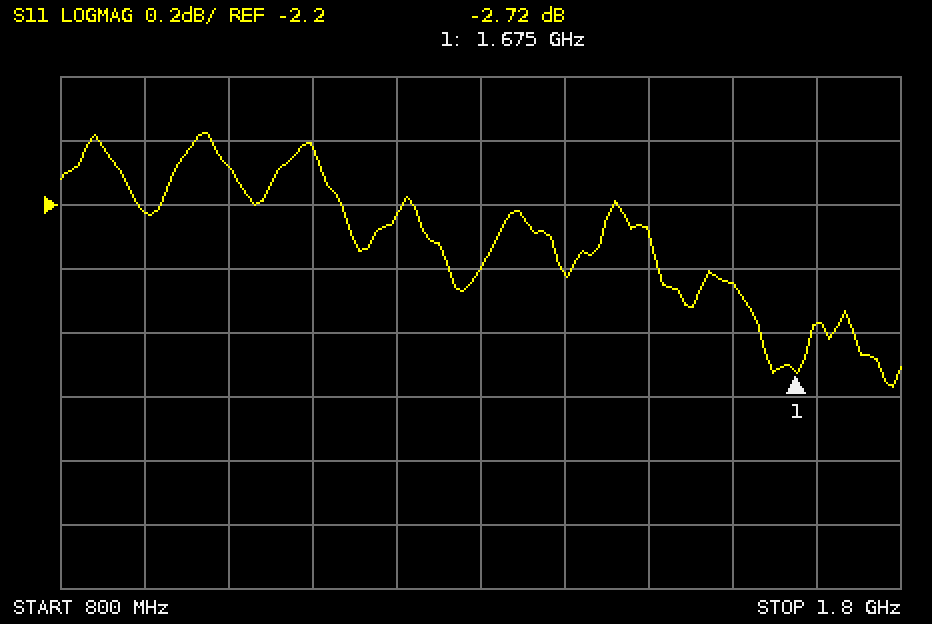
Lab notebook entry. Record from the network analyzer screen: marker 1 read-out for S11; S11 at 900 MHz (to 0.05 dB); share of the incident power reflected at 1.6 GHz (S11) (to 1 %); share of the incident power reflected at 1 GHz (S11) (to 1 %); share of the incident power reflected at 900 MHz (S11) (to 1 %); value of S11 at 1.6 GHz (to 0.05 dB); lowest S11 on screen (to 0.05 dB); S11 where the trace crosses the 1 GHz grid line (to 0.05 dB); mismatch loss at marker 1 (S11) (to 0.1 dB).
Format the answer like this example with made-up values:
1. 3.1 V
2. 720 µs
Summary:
1. -2.72 dB
2. -2.20 dB
3. 57 %
4. 62 %
5. 60 %
6. -2.45 dB
7. -2.75 dB
8. -2.10 dB
9. 3.3 dB
